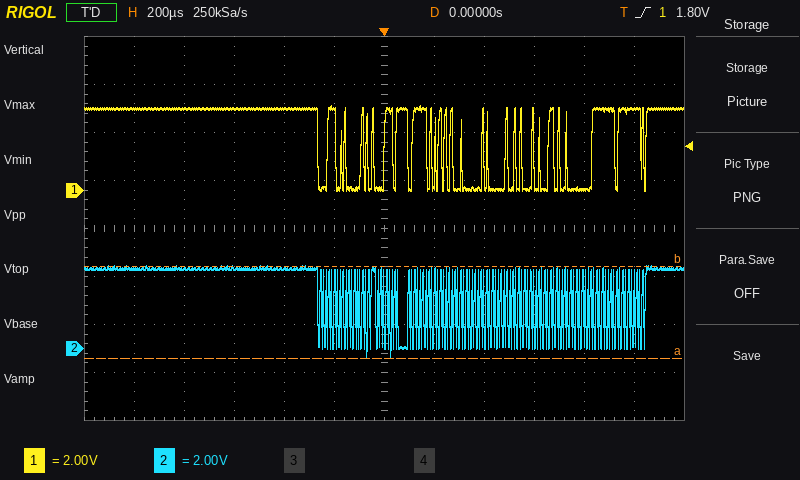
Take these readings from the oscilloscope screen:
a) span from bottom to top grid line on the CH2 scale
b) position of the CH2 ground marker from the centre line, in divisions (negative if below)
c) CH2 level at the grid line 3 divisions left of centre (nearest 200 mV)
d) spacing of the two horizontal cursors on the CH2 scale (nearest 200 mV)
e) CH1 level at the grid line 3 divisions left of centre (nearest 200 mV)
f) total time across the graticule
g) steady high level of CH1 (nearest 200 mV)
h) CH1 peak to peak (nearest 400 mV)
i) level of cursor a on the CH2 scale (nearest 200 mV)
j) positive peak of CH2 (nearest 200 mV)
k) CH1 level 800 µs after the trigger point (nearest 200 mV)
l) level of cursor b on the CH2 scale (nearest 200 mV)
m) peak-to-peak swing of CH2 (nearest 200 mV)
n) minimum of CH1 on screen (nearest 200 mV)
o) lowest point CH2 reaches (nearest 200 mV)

16 V
-2.5 div
3.4 V
3.8 V
3.4 V
2.4 ms
3.4 V
3.6 V
-400 mV
3.4 V
0.0 V
3.4 V
3.8 V
0.0 V
-400 mV
